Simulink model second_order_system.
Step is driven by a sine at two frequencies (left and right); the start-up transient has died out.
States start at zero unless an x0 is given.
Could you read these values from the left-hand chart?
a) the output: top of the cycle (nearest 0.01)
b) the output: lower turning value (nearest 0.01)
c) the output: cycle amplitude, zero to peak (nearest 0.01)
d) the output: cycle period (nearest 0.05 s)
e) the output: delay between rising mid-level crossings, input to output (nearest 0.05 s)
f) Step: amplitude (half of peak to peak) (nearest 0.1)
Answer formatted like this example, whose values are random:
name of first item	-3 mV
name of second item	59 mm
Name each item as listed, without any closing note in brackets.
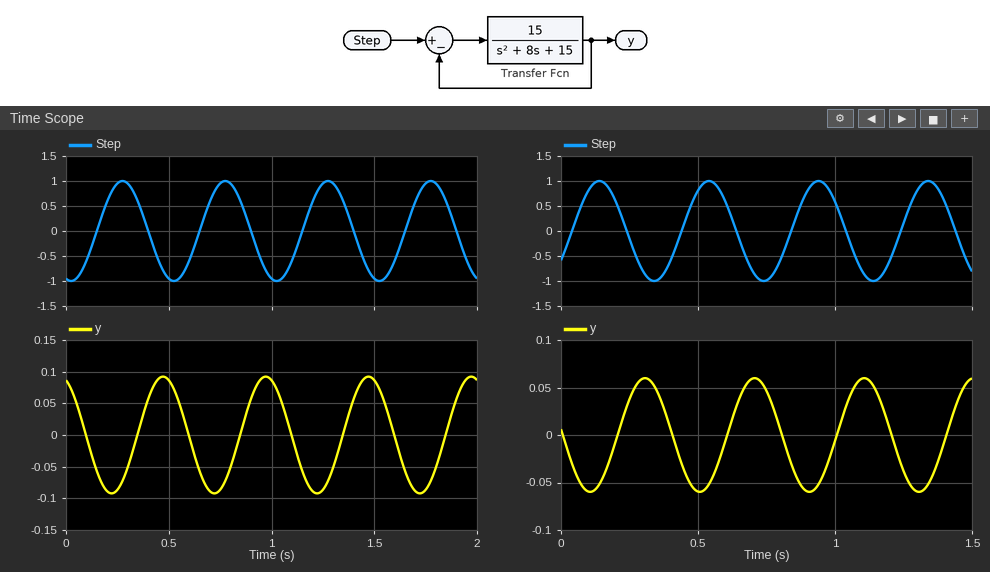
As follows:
the output: top of the cycle	0.09
the output: lower turning value	-0.09
the output: cycle amplitude, zero to peak	0.09
the output: cycle period	0.50 s
the output: delay between rising mid-level crossings, input to output	0.20 s
Step: amplitude (half of peak to peak)	1.0
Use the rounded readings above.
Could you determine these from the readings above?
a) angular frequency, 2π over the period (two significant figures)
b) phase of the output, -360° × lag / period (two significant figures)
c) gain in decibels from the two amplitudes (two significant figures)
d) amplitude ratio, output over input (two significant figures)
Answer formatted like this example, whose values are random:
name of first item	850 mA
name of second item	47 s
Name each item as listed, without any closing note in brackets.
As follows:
angular frequency, 2π over the period	13 rad/s
phase of the output, -360° × lag / period	-140°
gain in decibels from the two amplitudes	-21 dB
amplitude ratio, output over input	0.090
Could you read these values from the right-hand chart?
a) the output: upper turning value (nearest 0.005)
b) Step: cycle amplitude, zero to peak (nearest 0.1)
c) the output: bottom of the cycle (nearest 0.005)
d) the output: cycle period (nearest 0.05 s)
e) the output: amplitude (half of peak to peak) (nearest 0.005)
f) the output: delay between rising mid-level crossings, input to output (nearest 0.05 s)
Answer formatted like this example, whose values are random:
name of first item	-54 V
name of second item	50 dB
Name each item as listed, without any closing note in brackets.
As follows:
the output: upper turning value	0.060
Step: cycle amplitude, zero to peak	1.0
the output: bottom of the cycle	-0.060
the output: cycle period	0.40 s
the output: amplitude (half of peak to peak)	0.060
the output: delay between rising mid-level crossings, input to output	0.15 s
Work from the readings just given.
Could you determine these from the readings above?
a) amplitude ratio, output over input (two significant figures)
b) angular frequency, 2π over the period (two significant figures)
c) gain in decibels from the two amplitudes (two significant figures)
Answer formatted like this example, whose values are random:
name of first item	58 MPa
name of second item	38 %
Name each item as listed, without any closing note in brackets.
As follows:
amplitude ratio, output over input	0.060
angular frequency, 2π over the period	16 rad/s
gain in decibels from the two amplitudes	-24 dB
